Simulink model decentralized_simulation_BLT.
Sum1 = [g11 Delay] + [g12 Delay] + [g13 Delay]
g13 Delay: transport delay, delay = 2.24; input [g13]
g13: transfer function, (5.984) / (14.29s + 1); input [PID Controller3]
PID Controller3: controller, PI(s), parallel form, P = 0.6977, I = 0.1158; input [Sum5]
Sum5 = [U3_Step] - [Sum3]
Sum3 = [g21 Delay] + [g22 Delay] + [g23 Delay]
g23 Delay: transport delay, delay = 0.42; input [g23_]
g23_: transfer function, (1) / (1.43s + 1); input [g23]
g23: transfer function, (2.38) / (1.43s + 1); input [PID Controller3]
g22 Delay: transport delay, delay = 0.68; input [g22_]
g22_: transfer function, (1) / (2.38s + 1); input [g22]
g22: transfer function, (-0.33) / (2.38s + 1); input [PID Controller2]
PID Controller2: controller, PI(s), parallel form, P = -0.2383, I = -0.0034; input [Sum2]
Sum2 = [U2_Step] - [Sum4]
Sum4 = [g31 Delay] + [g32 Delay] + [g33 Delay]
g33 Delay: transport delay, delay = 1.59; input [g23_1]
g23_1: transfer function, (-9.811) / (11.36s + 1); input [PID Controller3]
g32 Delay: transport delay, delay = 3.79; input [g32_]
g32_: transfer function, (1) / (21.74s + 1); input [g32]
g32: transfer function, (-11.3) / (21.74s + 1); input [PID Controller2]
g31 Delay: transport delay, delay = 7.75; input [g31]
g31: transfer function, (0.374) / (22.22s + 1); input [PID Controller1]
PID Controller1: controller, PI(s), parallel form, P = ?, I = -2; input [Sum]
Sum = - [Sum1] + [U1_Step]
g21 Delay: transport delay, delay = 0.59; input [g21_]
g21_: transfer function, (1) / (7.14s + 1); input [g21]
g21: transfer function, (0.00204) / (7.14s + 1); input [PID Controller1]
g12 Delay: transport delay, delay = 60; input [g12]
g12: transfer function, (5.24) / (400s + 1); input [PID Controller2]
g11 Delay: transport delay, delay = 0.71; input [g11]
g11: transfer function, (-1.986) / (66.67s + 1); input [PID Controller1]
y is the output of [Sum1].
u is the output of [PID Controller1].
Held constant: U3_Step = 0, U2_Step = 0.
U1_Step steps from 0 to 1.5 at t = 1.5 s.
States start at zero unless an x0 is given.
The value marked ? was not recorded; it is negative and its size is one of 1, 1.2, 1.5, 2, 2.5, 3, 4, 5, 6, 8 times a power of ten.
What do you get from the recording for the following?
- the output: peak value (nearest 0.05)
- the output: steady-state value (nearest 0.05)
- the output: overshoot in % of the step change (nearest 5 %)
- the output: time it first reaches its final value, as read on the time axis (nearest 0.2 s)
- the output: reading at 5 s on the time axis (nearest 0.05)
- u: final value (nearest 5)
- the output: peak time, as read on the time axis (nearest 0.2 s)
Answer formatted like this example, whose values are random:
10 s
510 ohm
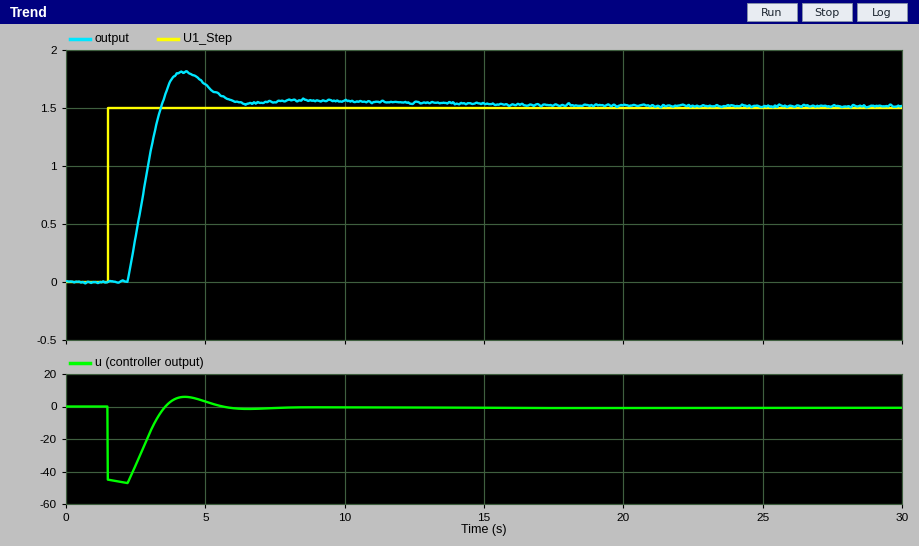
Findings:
1.80
1.50
20 %
3.4 s
1.70
0
4.2 s
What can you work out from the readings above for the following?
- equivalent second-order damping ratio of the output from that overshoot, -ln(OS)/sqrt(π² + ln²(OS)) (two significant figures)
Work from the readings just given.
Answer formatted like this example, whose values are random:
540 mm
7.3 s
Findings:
0.46
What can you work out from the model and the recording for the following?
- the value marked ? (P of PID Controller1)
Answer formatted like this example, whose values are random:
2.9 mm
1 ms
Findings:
-30
